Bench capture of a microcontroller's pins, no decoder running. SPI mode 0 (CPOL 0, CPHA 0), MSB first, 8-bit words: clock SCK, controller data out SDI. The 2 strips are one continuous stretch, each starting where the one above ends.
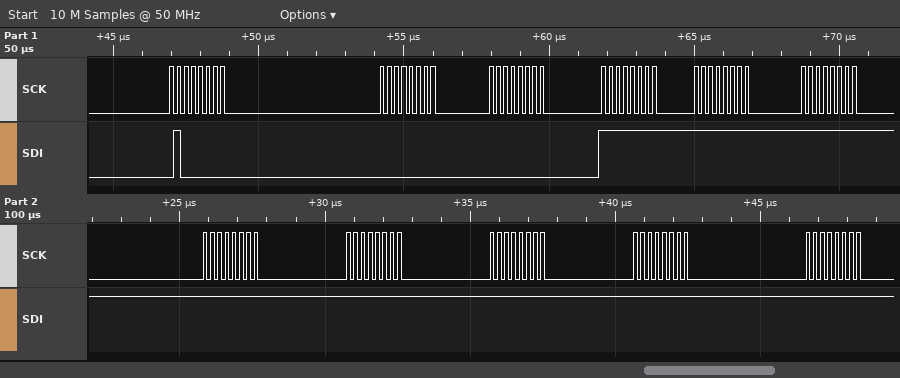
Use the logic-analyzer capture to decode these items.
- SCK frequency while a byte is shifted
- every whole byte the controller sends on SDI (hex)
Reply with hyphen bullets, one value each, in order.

- 4 MHz
- 0x40 0x00 0x00 0xFF 0xFF 0xFF 0xFF 0xFF 0xFF 0xFF 0xFF
